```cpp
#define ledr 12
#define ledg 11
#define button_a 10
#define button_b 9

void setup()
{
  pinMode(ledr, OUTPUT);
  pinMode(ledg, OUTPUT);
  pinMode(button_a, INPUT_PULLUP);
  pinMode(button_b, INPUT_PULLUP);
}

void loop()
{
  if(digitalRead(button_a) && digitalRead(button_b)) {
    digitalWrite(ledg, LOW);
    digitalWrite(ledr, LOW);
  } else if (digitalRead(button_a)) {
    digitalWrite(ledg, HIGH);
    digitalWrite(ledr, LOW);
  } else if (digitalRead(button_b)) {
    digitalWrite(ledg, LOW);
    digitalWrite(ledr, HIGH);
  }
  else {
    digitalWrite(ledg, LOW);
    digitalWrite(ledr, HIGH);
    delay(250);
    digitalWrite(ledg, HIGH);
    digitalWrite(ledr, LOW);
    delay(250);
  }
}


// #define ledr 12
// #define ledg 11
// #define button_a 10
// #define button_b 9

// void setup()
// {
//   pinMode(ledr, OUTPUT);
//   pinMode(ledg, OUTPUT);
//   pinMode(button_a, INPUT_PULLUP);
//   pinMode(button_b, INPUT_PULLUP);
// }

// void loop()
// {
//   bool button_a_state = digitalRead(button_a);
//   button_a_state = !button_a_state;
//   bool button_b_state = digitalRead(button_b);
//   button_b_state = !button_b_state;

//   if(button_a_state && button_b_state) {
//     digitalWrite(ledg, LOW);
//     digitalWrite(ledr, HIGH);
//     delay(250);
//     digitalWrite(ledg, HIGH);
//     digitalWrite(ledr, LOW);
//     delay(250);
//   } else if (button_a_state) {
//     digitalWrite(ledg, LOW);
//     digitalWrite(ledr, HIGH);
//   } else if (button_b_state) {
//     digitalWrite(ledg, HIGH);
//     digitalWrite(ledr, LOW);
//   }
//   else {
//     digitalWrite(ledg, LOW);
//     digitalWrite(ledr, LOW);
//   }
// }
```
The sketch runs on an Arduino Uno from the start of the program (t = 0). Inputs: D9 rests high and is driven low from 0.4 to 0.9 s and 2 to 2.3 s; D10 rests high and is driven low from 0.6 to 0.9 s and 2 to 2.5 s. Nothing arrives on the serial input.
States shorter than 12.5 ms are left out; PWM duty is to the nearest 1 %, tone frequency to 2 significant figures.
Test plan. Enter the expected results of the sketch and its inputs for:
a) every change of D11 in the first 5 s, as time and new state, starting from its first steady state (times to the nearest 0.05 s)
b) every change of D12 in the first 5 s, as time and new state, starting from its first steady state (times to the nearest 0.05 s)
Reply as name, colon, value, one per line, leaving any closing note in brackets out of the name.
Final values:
every change of D11 in the first 5 s, as time and new state, starting from its first steady state: 0 s low; 0.4 s high; 0.6 s low; 0.85 s high; 1.1 s low; 2.25 s high; 2.5 s low
every change of D12 in the first 5 s, as time and new state, starting from its first steady state: 0 s low; 0.6 s high; 0.85 s low; 2 s high; 2.25 s low
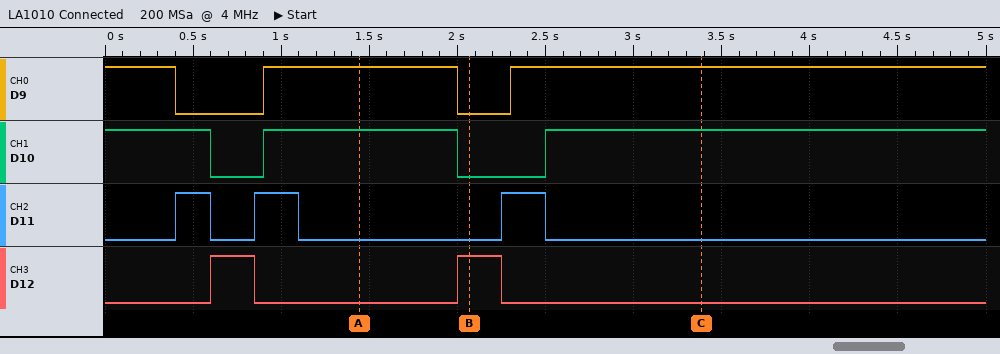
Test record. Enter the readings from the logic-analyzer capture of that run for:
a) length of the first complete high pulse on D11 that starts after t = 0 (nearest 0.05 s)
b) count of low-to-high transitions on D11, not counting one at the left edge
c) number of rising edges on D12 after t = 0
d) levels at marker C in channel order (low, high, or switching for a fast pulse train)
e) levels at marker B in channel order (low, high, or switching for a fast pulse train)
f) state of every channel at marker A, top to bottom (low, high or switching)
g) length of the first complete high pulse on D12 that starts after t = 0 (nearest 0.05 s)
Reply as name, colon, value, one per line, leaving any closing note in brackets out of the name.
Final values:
length of the first complete high pulse on D11 that starts after t = 0: 0.20 s
count of low-to-high transitions on D11, not counting one at the left edge: 3
number of rising edges on D12 after t = 0: 2
levels at marker C in channel order: D9 high, D10 high, D11 low, D12 low
levels at marker B in channel order: D9 low, D10 low, D11 low, D12 high
state of every channel at marker A, top to bottom: D9 high, D10 high, D11 low, D12 low
length of the first complete high pulse on D12 that starts after t = 0: 0.25 s
